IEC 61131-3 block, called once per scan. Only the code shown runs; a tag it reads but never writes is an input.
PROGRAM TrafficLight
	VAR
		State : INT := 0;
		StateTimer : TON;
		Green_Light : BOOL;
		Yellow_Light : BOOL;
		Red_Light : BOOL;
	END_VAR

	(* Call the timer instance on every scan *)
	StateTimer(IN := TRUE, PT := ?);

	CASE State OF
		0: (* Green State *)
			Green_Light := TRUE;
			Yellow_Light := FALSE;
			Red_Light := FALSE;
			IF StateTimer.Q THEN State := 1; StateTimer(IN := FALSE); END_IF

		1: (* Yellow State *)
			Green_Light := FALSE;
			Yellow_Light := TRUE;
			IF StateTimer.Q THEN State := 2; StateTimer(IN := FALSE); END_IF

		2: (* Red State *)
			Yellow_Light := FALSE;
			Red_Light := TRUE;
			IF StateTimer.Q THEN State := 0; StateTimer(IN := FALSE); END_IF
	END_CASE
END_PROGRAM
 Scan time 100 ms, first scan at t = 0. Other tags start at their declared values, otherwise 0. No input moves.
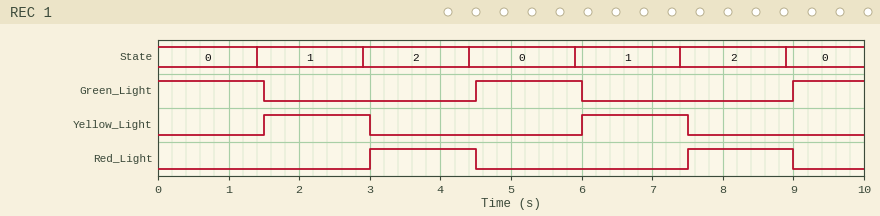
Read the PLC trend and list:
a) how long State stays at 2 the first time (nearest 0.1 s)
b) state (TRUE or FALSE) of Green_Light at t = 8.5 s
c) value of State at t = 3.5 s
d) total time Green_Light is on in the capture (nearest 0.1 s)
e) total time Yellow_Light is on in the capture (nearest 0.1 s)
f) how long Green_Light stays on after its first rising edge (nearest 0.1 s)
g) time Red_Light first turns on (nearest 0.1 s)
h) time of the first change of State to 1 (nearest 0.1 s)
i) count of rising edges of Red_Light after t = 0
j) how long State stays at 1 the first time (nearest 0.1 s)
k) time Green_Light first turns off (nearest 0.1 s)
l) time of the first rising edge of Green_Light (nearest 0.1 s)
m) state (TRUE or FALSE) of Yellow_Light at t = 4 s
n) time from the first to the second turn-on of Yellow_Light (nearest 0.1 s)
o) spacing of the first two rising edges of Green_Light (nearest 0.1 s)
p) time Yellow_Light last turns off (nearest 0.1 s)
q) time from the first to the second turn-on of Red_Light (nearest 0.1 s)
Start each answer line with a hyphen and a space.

- 1.5 s
- FALSE
- 2
- 4.0 s
- 3.0 s
- 1.5 s
- 3.0 s
- 1.4 s
- 2
- 1.5 s
- 1.5 s
- 4.5 s
- FALSE
- 4.5 s
- 4.5 s
- 7.5 s
- 4.5 s
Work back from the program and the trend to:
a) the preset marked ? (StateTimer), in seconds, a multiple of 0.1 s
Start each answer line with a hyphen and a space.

- 1.4 s
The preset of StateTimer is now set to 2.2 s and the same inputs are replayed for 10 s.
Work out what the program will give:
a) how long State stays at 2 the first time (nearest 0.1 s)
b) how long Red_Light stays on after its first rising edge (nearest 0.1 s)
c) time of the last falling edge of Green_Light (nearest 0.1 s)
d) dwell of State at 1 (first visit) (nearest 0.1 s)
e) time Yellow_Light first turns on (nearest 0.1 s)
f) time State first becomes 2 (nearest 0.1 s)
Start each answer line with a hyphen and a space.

- 2.3 s
- 2.3 s
- 9.2 s
- 2.3 s
- 2.3 s
- 4.5 s
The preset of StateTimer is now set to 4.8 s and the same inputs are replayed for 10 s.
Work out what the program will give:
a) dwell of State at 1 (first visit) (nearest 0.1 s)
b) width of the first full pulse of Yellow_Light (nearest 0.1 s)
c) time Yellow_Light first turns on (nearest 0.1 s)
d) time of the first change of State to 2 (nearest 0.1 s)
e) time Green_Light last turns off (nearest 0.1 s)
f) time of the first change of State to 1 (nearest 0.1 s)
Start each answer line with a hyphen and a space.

- 4.9 s
- 4.9 s
- 4.9 s
- 9.7 s
- 4.9 s
- 4.8 s
